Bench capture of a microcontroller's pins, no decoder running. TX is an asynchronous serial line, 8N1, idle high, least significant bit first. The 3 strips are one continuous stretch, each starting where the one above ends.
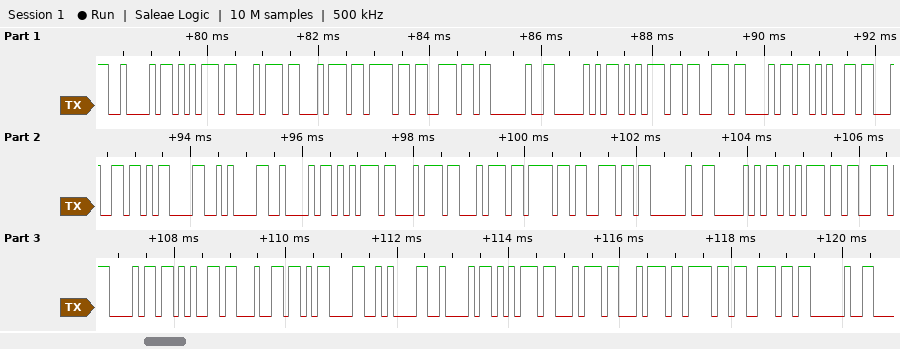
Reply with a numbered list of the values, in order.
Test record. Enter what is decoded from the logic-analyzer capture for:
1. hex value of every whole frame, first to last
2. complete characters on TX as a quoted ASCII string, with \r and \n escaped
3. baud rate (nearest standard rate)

1. 0x42 0x75 0x74 0x74 0x6F 0x6E 0x20 0x50 0x75 0x73 0x68 0x65 0x64 0x0D 0x0A 0x42 0x75 0x74 0x74 0x6F 0x6E 0x20 0x50 0x75 0x73 0x68 0x65 0x64 0x0D 0x0A 0x42 0x75 0x74 0x74 0x6F 0x6E 0x20
2. "Button Pushed\r\nButton Pushed\r\nButton "
3. 9600 baud
